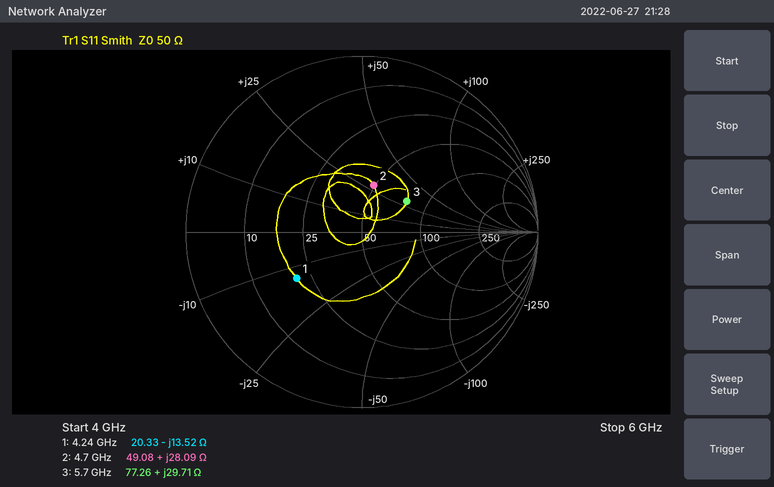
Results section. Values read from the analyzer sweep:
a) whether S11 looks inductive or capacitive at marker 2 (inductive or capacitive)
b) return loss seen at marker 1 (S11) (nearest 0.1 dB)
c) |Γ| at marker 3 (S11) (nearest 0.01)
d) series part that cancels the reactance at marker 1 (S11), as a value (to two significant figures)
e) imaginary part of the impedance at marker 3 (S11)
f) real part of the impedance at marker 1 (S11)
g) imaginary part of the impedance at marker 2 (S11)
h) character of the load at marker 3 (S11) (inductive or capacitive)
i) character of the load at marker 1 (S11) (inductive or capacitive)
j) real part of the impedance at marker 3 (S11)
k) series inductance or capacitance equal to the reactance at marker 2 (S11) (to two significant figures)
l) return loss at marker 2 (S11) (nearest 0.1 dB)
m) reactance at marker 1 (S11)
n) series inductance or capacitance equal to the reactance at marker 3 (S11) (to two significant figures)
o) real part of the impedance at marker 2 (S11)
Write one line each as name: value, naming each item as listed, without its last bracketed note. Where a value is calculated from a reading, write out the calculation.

whether S11 looks inductive or capacitive at marker 2: inductive
return loss seen at marker 1 (S11): 6.8 dB
|Γ| at marker 3 (S11): 0.31
series part that cancels the reactance at marker 1 (S11), as a value: L = 13.52 Ω/(2π × 4.24 GHz) ≈ 507 pH, so 510 pH to two significant figures
imaginary part of the impedance at marker 3: +29.71 Ω
real part of the impedance at marker 1: 20.33 Ω
imaginary part of the impedance at marker 2: +28.09 Ω
character of the load at marker 3 (S11): inductive
character of the load at marker 1 (S11): capacitive
real part of the impedance at marker 3: 77.26 Ω
series inductance or capacitance equal to the reactance at marker 2 (S11): L = 28.09 Ω/(2π × 4.7 GHz) ≈ 951 pH, so 950 pH to two significant figures
return loss at marker 2 (S11): 11.3 dB
reactance at marker 1: -13.52 Ω
series inductance or capacitance equal to the reactance at marker 3 (S11): L = 29.71 Ω/(2π × 5.7 GHz) ≈ 830 pH
real part of the impedance at marker 2: 49.08 Ω
